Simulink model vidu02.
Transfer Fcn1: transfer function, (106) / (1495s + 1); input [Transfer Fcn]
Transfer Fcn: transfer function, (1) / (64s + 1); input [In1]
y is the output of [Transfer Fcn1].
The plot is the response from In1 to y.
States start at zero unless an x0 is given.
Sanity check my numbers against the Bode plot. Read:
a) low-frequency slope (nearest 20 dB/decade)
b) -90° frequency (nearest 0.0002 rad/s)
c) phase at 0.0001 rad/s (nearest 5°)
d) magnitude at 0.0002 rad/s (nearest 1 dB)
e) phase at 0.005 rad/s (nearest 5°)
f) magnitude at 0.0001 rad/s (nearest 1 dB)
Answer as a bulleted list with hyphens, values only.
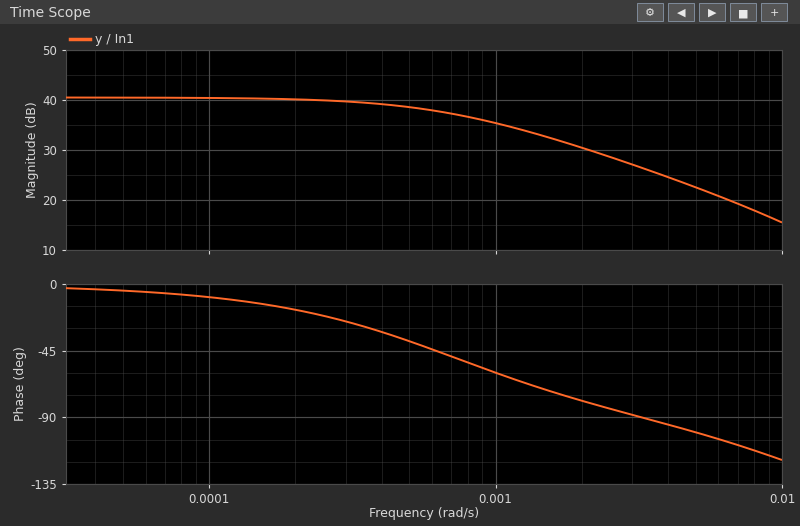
- 0 dB/decade
- 0.0032 rad/s
- -10°
- 40 dB
- -100°
- 40 dB
